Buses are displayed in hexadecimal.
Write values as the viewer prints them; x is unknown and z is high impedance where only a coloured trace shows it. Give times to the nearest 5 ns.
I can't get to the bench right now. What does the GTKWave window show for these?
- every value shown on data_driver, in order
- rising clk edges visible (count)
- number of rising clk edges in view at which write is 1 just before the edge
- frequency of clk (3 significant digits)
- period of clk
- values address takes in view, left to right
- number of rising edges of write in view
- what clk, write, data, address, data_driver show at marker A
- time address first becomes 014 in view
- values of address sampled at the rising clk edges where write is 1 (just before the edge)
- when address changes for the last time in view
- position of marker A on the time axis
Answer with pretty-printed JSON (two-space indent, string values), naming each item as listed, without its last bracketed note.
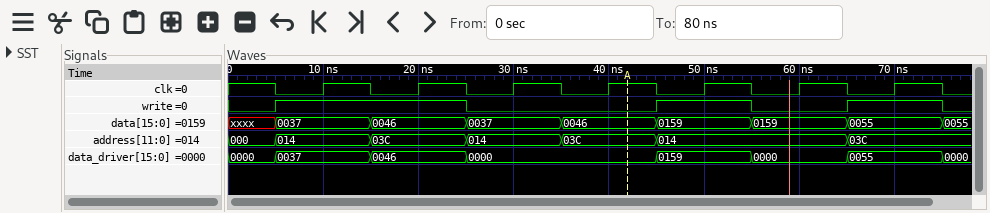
{
  "every value shown on data_driver, in order": "0000, 0037, 0046, 0000, 0159, 0000, 0055, 0000",
  "rising clk edges visible": "7",
  "number of rising clk edges in view at which write is 1 just before the edge": "4",
  "frequency of clk": "100 MHz",
  "period of clk": "10 ns",
  "values address takes in view, left to right": "000, 014, 03C, 014, 03C, 014, 03C",
  "number of rising edges of write in view": "3",
  "what clk, write, data, address, data_driver show at marker A": "clk=1, write=0, data=0046, address=03C, data_driver=0000",
  "time address first becomes 014 in view": "5 ns",
  "values of address sampled at the rising clk edges where write is 1": "014, 03C, 014, 03C",
  "when address changes for the last time in view": "65 ns",
  "position of marker A on the time axis": "40 ns"
}
